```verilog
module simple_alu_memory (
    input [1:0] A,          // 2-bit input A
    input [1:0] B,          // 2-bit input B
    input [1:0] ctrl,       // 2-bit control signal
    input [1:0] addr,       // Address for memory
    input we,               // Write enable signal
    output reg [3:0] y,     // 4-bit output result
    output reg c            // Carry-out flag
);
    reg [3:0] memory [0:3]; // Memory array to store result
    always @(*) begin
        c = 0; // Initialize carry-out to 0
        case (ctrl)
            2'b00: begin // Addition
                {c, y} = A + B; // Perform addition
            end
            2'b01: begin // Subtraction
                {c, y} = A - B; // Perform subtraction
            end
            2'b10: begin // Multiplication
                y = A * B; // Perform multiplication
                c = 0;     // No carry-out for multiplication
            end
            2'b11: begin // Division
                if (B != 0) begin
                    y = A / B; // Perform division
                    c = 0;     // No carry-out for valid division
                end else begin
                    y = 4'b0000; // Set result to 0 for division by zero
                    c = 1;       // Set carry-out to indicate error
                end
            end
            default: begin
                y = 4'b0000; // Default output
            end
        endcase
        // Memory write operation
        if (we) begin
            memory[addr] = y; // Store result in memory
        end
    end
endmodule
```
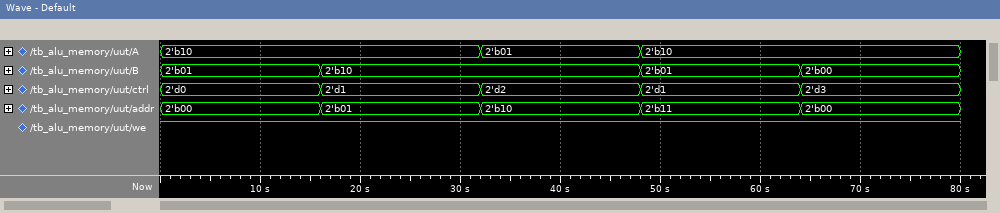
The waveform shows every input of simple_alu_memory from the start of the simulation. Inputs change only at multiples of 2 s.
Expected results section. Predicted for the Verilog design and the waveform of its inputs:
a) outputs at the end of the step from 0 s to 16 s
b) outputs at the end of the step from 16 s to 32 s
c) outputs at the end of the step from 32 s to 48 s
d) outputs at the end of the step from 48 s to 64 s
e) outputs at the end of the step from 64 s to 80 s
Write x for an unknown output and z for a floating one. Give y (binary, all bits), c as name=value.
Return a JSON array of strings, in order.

["y=0011, c=0", "y=0000, c=0", "y=0010, c=0", "y=0001, c=0", "y=0000, c=1"]
